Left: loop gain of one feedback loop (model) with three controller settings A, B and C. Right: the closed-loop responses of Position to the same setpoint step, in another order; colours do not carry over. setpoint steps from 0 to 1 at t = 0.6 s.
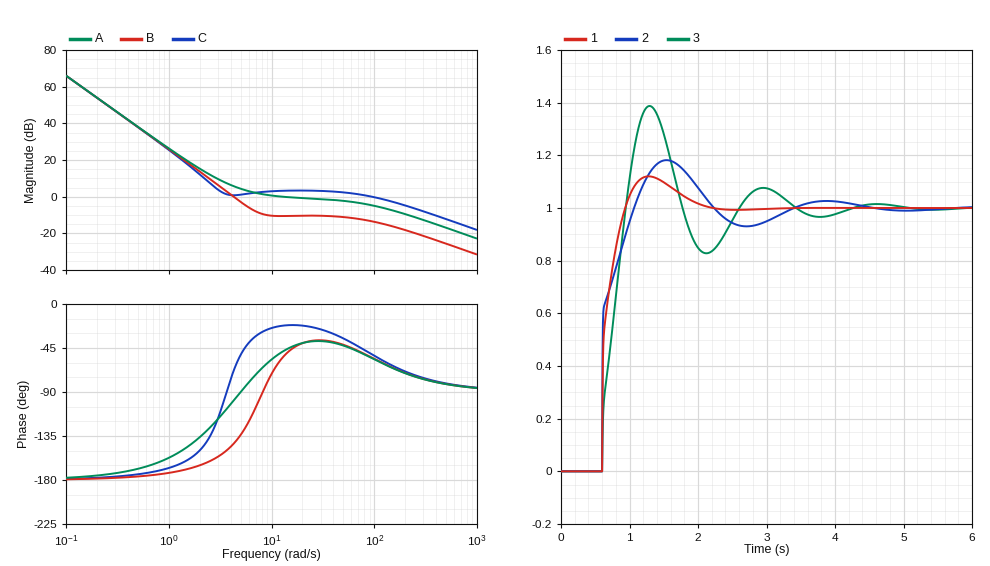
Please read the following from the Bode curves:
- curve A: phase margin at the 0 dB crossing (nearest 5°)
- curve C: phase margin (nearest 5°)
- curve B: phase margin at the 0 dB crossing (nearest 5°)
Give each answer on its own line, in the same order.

130°
130°
35°
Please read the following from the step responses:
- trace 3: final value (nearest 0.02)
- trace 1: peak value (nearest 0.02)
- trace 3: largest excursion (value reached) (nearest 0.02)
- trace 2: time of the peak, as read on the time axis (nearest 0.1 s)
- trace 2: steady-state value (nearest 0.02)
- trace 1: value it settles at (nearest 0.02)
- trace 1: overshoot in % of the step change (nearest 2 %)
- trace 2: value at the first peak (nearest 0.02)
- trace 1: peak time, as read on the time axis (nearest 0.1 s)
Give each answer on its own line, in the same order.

1.00
1.12
1.38
1.5 s
1.00
1.00
12 %
1.18
1.3 s
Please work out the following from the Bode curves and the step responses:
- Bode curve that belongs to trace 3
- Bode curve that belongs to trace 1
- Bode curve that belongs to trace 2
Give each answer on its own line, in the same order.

B
A
C
